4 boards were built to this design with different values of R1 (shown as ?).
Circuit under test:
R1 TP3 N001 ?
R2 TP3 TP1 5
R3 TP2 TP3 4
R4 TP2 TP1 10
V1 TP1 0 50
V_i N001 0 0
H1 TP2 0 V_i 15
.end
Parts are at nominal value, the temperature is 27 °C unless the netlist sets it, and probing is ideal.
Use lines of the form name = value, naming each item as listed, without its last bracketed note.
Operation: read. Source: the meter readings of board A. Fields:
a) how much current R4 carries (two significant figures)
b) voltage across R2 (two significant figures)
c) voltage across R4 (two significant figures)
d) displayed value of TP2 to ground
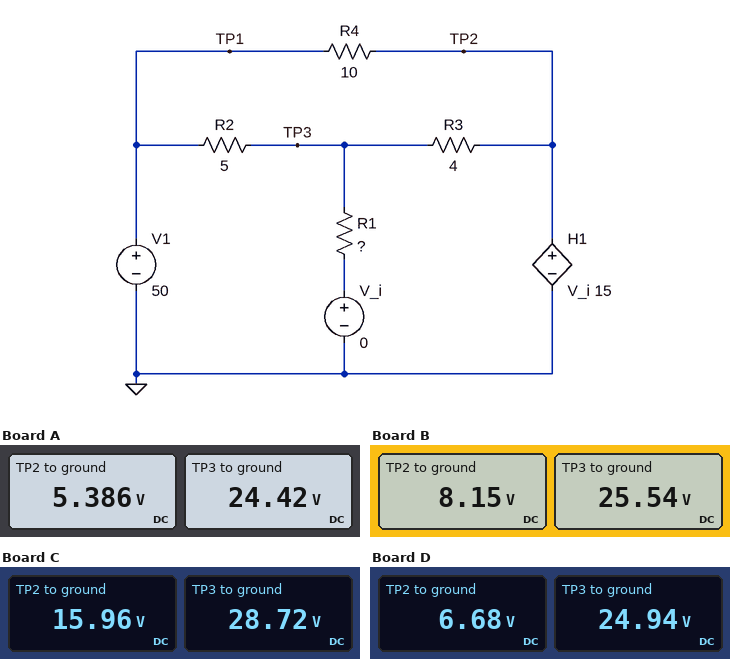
how much current R4 carries = 4.5 A
voltage across R2 = 26 V
voltage across R4 = 45 V
displayed value of TP2 to ground = 5.386 V
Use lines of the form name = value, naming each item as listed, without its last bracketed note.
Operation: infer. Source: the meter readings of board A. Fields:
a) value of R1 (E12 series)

value of R1 = 68 Ω
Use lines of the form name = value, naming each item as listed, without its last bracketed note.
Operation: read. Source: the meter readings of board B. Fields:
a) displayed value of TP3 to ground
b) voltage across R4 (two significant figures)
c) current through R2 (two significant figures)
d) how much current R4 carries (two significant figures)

displayed value of TP3 to ground = 25.54 V
voltage across R4 = 42 V
current through R2 = 4.9 A
how much current R4 carries = 4.2 A
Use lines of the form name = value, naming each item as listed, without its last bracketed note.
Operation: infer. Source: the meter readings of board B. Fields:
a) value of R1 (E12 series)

value of R1 = 47 Ω
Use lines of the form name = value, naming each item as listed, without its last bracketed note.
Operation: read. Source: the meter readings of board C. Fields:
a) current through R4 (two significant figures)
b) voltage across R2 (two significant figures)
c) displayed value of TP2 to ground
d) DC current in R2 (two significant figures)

current through R4 = 3.4 A
voltage across R2 = 21 V
displayed value of TP2 to ground = 15.96 V
DC current in R2 = 4.3 A
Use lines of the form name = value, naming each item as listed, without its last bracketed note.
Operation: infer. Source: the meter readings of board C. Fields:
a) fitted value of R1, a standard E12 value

fitted value of R1, a standard E12 value = 27 Ω
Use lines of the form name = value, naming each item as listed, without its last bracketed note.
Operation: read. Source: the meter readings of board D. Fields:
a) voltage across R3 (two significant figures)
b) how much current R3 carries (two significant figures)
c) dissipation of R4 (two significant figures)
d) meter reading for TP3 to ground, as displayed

voltage across R3 = 18 V
how much current R3 carries = 4.6 A
dissipation of R4 = 190 W
meter reading for TP3 to ground, as displayed = 24.94 V
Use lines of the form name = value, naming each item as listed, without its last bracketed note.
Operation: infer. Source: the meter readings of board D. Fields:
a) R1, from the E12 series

R1, from the E12 series = 56 Ω
